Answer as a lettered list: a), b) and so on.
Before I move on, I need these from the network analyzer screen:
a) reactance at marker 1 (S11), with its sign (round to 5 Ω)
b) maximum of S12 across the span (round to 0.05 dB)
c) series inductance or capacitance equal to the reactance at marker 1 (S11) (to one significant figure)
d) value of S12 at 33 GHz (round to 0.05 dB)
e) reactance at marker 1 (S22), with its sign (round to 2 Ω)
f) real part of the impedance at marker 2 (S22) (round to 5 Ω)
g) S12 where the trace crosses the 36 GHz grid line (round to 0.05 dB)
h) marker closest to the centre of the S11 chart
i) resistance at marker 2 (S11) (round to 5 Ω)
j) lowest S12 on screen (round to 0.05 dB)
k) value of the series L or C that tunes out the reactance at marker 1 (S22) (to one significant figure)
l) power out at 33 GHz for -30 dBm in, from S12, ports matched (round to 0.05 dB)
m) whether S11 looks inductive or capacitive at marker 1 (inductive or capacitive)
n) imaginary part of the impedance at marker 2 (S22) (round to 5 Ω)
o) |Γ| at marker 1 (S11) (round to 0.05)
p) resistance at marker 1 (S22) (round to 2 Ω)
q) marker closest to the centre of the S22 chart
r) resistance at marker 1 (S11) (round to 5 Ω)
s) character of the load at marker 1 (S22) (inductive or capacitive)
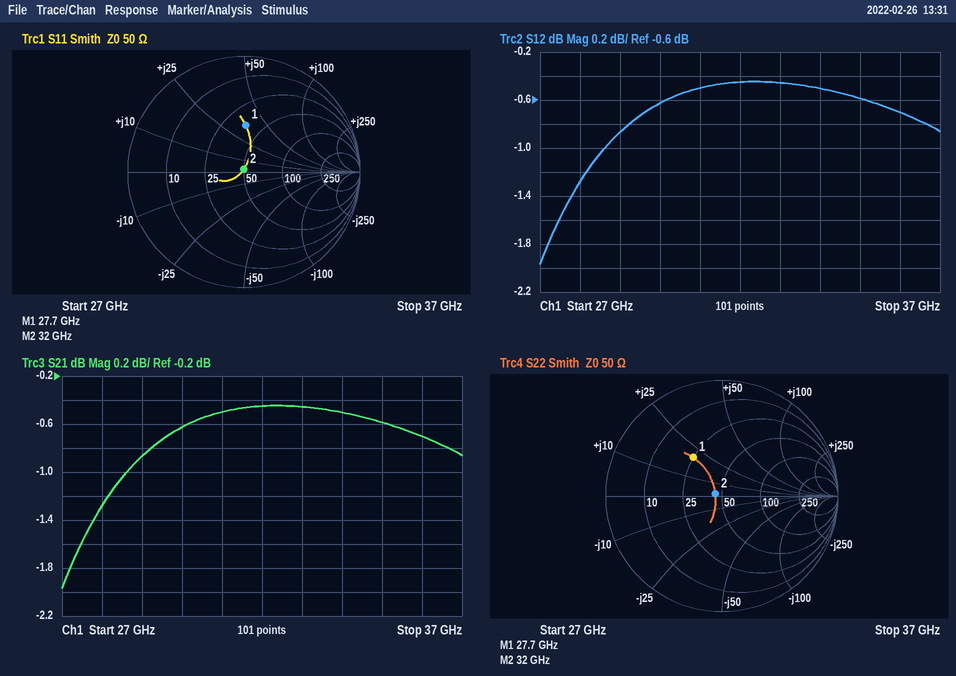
a) +35 Ω
b) -0.45 dB
c) 200 pH
d) -0.45 dB
e) +20 Ω
f) 45 Ω
g) -0.70 dB
h) marker 2
i) 50 Ω
j) -1.95 dB
k) 300 fF
l) -30.45 dBm
m) inductive
n) 0 Ω
o) 0.40
p) 24 Ω
q) marker 2
r) 35 Ω
s) inductive
